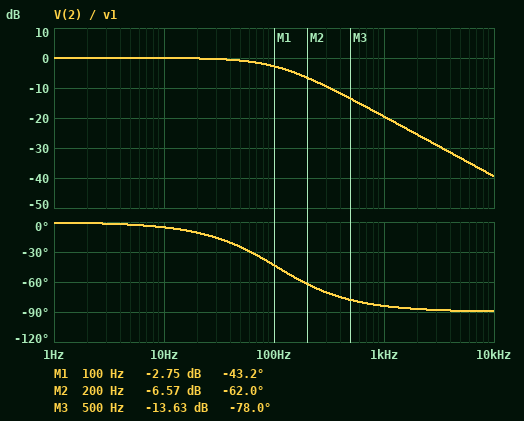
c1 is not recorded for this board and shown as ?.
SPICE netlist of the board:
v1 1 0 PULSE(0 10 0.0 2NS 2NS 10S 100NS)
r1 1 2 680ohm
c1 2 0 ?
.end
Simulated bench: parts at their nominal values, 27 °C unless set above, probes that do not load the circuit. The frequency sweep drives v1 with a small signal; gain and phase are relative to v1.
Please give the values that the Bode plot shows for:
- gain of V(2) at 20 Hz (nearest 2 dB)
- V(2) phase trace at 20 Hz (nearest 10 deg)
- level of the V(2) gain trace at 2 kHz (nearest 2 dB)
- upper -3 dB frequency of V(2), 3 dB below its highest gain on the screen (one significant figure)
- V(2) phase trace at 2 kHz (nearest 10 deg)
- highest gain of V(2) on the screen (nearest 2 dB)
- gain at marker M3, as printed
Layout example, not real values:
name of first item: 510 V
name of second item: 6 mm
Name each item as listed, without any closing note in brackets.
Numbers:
gain of V(2) at 20 Hz: 0 dB
V(2) phase trace at 20 Hz: -10 deg
level of the V(2) gain trace at 2 kHz: -26 dB
upper -3 dB frequency of V(2), 3 dB below its highest gain on the screen: 100 Hz
V(2) phase trace at 2 kHz: -90 deg
highest gain of V(2) on the screen: 0 dB
gain at marker M3, as printed: -13.63 dB
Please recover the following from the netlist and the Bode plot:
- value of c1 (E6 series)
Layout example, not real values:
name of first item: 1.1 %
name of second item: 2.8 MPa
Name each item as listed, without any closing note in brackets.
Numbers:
value of c1: 2.2 µF
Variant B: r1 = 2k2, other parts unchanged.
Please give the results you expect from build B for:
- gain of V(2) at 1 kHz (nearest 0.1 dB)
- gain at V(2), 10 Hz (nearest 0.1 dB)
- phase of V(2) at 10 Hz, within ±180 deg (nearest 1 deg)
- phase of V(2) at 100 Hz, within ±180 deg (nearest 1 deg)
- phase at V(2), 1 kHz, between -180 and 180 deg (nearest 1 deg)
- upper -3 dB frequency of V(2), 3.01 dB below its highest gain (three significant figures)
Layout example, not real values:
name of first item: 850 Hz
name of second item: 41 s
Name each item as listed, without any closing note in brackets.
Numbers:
gain of V(2) at 1 kHz: -29.7 dB
gain at V(2), 10 Hz: -0.4 dB
phase of V(2) at 10 Hz, within ±180 deg: -17 deg
phase of V(2) at 100 Hz, within ±180 deg: -72 deg
phase at V(2), 1 kHz, between -180 and 180 deg: -88 deg
upper -3 dB frequency of V(2), 3.01 dB below its highest gain: 32.9 Hz
